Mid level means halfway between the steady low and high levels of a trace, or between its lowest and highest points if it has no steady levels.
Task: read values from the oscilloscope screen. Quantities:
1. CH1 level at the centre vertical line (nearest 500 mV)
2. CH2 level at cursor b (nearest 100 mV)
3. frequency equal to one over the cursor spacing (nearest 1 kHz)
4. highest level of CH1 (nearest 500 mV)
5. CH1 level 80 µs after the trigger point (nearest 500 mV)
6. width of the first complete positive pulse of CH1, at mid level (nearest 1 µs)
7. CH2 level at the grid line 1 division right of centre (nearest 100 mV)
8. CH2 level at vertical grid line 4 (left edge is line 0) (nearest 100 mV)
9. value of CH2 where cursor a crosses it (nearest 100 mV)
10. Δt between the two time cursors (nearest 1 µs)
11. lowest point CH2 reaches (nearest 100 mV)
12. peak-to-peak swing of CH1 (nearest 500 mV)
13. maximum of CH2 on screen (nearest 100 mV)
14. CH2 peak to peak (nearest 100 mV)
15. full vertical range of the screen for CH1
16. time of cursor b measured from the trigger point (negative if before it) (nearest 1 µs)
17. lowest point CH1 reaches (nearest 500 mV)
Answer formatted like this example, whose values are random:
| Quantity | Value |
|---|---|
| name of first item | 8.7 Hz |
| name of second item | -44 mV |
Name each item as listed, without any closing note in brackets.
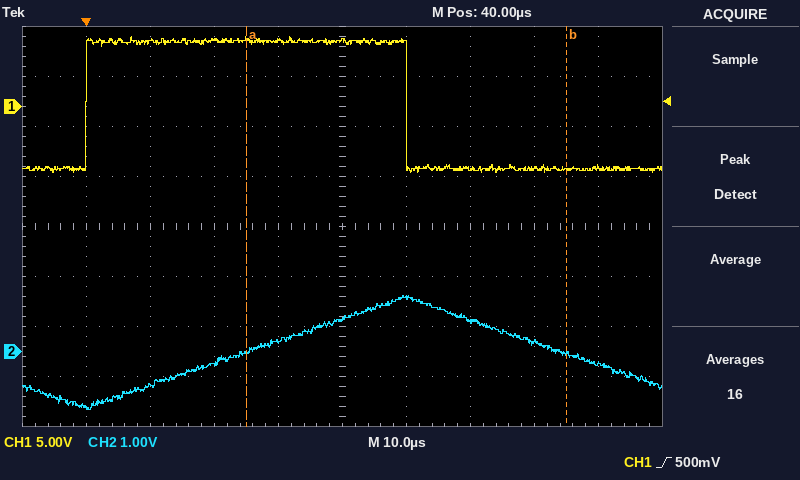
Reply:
| Quantity | Value |
|---|---|
| CH1 level at the centre vertical line | 6.5 V |
| CH2 level at cursor b | -100 mV |
| frequency equal to one over the cursor spacing | 20 kHz |
| highest level of CH1 | 7.0 V |
| CH1 level 80 µs after the trigger point | -6.0 V |
| width of the first complete positive pulse of CH1, at mid level | 50 µs |
| CH2 level at the grid line 1 division right of centre | 1.1 V |
| CH2 level at vertical grid line 4 (left edge is line 0) | 200 mV |
| value of CH2 where cursor a crosses it | 0.0 V |
| Δt between the two time cursors | 50 µs |
| lowest point CH2 reaches | -1.2 V |
| peak-to-peak swing of CH1 | 13.5 V |
| maximum of CH2 on screen | 1.1 V |
| CH2 peak to peak | 2.3 V |
| full vertical range of the screen for CH1 | 40 V |
| time of cursor b measured from the trigger point (negative if before it) | +75 µs |
| lowest point CH1 reaches | -6.5 V |
